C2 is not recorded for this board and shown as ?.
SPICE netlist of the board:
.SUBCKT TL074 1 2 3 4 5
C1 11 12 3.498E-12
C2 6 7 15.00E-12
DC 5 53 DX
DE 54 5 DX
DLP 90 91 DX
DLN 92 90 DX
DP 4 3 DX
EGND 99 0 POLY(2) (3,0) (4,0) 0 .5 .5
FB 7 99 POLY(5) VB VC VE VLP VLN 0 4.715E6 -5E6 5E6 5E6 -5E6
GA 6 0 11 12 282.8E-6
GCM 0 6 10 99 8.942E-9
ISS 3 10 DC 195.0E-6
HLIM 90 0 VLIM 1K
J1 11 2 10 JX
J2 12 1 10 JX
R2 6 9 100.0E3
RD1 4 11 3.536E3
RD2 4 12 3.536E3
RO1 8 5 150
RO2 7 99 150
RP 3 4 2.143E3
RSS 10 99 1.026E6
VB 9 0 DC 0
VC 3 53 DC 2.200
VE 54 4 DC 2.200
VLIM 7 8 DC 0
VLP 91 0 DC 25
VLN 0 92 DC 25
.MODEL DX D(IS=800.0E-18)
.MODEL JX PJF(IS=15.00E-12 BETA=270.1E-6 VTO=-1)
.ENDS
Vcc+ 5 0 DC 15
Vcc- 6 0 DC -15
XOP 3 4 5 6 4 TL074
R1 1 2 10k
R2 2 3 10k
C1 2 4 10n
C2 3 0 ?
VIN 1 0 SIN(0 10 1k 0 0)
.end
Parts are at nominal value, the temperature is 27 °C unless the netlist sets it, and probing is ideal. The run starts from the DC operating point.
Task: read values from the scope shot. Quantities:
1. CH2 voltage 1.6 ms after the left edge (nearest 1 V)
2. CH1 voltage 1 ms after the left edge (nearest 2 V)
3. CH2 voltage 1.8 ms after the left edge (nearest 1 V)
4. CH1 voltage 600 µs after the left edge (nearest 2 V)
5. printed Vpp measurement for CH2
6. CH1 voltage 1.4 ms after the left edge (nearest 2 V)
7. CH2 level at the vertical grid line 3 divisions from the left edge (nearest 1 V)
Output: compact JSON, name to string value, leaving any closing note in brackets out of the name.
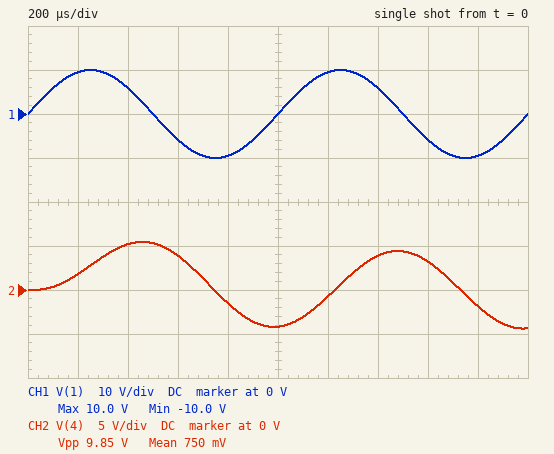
{"CH2 voltage 1.6 ms after the left edge": "3 V", "CH1 voltage 1 ms after the left edge": "0 V", "CH2 voltage 1.8 ms after the left edge": "-2 V", "CH1 voltage 600 µs after the left edge": "-6 V", "printed Vpp measurement for CH2": "9.85 V", "CH1 voltage 1.4 ms after the left edge": "6 V", "CH2 level at the vertical grid line 3 divisions from the left edge": "4 V"}
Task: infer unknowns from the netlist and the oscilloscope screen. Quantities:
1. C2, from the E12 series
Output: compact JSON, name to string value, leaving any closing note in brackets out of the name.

{"C2, from the E12 series": "18 nF"}
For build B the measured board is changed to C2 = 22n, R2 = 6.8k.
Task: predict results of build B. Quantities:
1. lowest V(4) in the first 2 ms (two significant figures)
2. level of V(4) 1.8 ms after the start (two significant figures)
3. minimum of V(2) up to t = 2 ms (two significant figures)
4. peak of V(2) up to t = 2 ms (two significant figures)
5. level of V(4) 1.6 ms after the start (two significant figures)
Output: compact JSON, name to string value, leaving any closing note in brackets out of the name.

{"lowest V(4) in the first 2 ms": "-4.2 V", "level of V(4) 1.8 ms after the start": "-2.0 V", "minimum of V(2) up to t = 2 ms": "-5.8 V", "peak of V(2) up to t = 2 ms": "6.7 V", "level of V(4) 1.6 ms after the start": "3.0 V"}
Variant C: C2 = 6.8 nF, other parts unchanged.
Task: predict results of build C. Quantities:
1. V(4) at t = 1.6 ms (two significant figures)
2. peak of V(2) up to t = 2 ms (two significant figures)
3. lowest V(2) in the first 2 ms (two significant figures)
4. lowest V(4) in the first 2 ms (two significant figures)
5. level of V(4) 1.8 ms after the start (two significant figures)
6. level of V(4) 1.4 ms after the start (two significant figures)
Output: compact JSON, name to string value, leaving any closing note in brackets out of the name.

{"V(4) at t = 1.6 ms": "2.1 V", "peak of V(2) up to t = 2 ms": "9.7 V", "lowest V(2) in the first 2 ms": "-9.7 V", "lowest V(4) in the first 2 ms": "-8.9 V", "level of V(4) 1.8 ms after the start": "-7.6 V", "level of V(4) 1.4 ms after the start": "8.9 V"}
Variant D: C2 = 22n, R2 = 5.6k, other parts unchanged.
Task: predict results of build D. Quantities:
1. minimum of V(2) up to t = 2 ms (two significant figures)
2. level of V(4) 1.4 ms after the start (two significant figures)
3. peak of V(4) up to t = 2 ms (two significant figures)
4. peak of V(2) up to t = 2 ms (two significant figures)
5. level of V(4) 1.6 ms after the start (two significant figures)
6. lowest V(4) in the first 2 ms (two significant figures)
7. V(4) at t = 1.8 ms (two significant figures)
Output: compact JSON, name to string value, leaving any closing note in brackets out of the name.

{"minimum of V(2) up to t = 2 ms": "-5.7 V", "level of V(4) 1.4 ms after the start": "4.2 V", "peak of V(4) up to t = 2 ms": "5.6 V", "peak of V(2) up to t = 2 ms": "6.6 V", "level of V(4) 1.6 ms after the start": "3.0 V", "lowest V(4) in the first 2 ms": "-4.5 V", "V(4) at t = 1.8 ms": "-2.3 V"}
